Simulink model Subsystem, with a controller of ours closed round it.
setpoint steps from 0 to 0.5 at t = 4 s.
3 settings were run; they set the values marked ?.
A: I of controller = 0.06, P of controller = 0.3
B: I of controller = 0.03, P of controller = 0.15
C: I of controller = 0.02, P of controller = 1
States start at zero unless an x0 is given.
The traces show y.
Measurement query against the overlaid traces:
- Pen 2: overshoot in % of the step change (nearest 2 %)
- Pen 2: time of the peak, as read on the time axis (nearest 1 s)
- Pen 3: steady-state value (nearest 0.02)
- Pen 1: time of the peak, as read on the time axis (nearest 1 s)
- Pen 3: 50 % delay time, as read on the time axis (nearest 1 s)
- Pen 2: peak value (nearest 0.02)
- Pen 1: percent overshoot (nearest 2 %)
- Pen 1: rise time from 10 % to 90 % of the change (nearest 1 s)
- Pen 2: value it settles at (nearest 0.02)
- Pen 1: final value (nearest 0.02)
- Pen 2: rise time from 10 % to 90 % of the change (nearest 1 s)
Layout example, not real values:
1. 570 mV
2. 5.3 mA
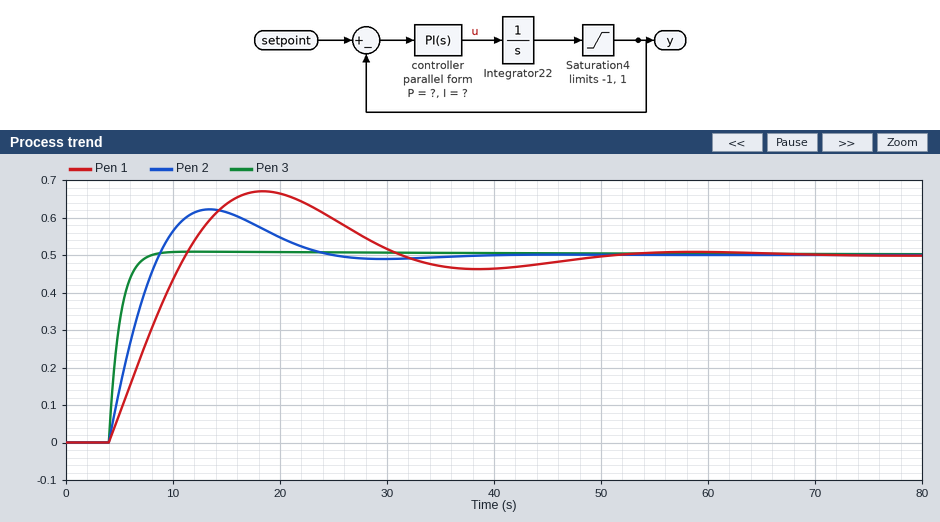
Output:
1. 24 %
2. 13 s
3. 0.50
4. 18 s
5. 5 s
6. 0.62
7. 34 %
8. 6 s
9. 0.50
10. 0.50
11. 4 s
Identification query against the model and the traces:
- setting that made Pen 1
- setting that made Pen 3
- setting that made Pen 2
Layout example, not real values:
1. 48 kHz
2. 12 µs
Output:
1. B
2. C
3. A
